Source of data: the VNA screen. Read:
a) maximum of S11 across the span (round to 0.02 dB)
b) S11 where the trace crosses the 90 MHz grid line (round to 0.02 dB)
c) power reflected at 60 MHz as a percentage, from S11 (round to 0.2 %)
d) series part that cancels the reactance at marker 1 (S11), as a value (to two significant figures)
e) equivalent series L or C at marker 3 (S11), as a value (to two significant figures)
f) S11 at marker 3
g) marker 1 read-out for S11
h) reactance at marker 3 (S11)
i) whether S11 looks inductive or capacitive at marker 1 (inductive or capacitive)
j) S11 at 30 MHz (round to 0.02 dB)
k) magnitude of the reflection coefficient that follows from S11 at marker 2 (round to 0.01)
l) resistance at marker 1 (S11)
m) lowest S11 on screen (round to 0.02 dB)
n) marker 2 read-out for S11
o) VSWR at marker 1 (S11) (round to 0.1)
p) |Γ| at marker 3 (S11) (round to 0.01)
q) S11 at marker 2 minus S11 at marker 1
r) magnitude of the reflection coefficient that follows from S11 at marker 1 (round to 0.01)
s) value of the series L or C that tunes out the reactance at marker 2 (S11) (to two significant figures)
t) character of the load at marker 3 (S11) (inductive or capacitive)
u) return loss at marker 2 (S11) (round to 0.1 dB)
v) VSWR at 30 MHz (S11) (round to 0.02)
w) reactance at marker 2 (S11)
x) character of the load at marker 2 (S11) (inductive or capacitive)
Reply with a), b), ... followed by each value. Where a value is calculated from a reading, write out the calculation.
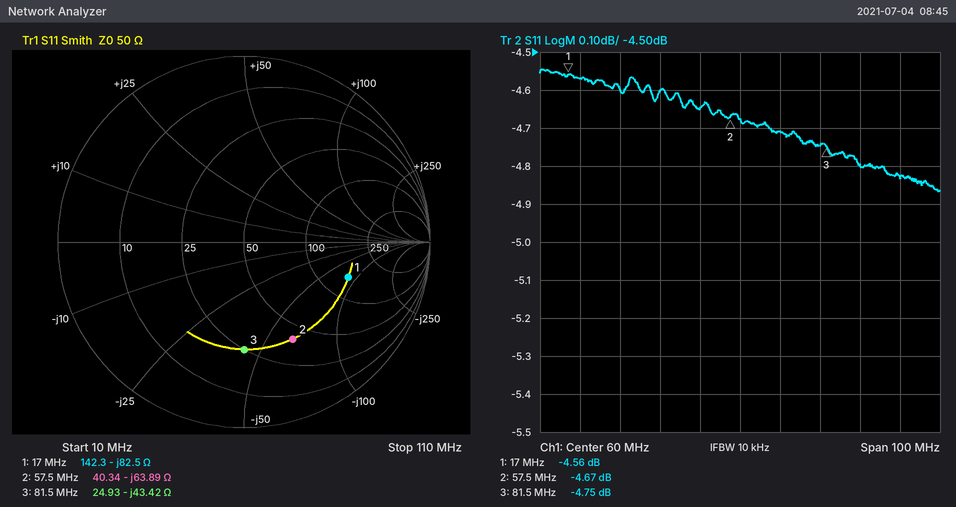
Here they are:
a) -4.54 dB
b) -4.80 dB
c) 10^(-4.68/10) ≈ 34.0 %
d) L = 82.5 Ω/(2π × 17 MHz) ≈ 772 nH, so 770 nH to two significant figures
e) C = 1/(2π × 81.5 MHz × 43.42 Ω) ≈ 45 pF
f) -4.75 dB
g) -4.56 dB
h) -43.42 Ω
i) capacitive
j) -4.60 dB
k) 10^(-4.67/20) ≈ 0.58
l) 142.3 Ω
m) -4.86 dB
n) -4.67 dB
o) 3.9
p) 0.58
q) -4.67 − (-4.56) = -0.11 dB
r) 10^(-4.56/20) ≈ 0.59
s) L = 63.89 Ω/(2π × 57.5 MHz) ≈ 177 nH, so 180 nH to two significant figures
t) capacitive
u) 4.7 dB
v) |Γ| = 10^(-4.6/20) = 0.5888; VSWR = (1 + 0.5888)/(1 − 0.5888) ≈ 3.86
w) -63.89 Ω
x) capacitive
